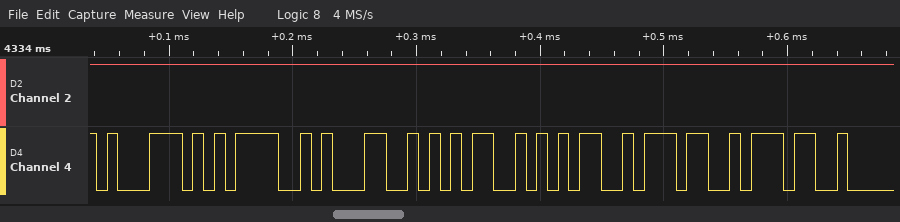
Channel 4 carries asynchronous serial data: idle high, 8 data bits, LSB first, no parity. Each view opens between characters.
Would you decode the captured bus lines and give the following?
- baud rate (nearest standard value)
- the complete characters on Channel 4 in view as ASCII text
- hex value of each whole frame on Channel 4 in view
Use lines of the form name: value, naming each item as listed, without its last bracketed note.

baud rate: 115200 baud
the complete characters on Channel 4 in view as ASCII text: "q=15577"
hex value of each whole frame on Channel 4 in view: 71, 3D, 31, 35, 35, 37, 37
